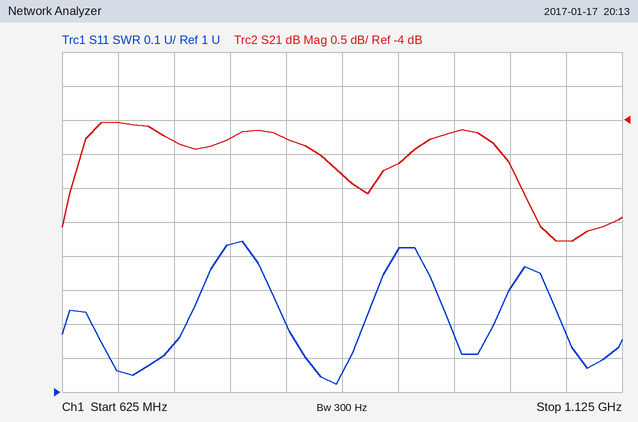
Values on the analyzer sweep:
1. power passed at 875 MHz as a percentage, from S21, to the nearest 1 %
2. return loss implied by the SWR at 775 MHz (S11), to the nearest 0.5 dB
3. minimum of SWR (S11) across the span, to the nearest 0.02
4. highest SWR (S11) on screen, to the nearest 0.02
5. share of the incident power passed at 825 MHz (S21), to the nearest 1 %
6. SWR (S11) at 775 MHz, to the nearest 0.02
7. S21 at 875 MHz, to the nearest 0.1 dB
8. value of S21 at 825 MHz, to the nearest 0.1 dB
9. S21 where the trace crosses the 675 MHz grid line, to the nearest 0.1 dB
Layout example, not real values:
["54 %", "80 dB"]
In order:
["33 %", "15.0 dB", "1.02", "1.44", "37 %", "1.44", "-4.8 dB", "-4.3 dB", "-4.0 dB"]
